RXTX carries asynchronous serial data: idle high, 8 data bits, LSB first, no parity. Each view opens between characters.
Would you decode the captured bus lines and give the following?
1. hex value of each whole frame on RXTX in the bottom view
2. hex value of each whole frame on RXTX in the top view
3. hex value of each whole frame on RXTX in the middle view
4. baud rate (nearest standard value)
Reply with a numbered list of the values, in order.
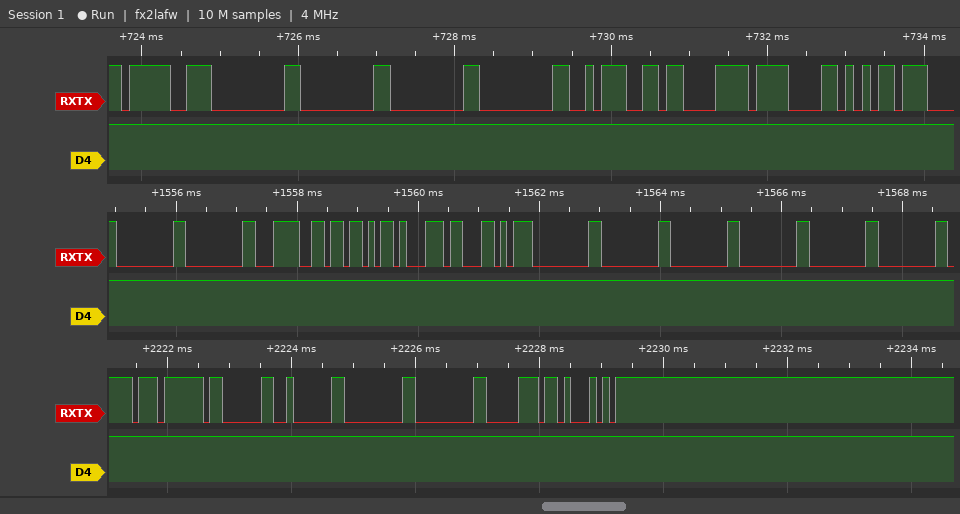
1. F7, 03, 02, 00, 00, 70, 51
2. 9F, 00, 00, 00, 00, 3A, C3, 0F, B5
3. 00, 00, 3C, 5B, 71, AC, 00, 00, 00, 00, 00, 00
4. 9600 baud
